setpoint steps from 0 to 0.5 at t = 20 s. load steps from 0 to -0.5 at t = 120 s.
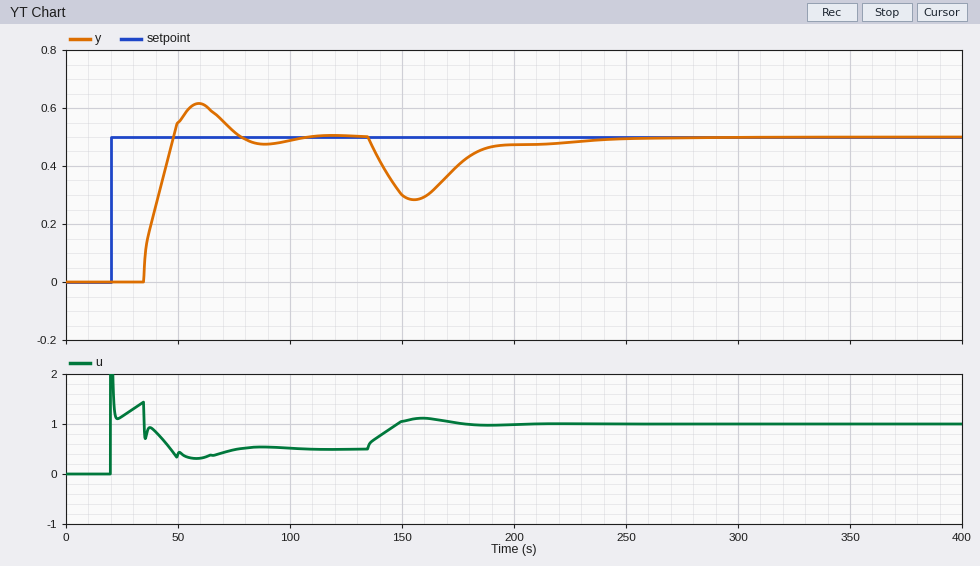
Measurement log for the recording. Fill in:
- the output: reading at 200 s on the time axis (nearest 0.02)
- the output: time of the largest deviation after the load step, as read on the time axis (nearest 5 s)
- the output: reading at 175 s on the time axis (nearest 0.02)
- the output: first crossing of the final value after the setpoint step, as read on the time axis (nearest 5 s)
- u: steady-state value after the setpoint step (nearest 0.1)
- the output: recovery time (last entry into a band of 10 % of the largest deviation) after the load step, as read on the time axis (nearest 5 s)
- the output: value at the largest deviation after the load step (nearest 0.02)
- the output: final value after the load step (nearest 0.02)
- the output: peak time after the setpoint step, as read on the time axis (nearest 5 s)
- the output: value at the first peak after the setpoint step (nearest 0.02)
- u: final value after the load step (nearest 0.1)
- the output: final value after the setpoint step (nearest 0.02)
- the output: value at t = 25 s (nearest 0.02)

0.48
155 s
0.40
50 s
0.5
220 s
0.28
0.50
60 s
0.62
1.0
0.50
0.00
